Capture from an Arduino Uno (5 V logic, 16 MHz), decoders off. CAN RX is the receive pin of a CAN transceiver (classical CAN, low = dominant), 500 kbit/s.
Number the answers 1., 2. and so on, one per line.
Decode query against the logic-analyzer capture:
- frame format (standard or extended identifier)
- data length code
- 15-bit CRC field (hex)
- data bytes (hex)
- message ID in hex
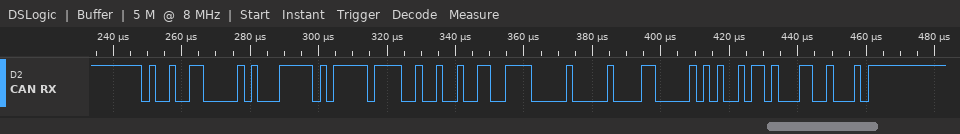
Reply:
1. standard
2. 8
3. 0x68C8
4. FD FF 24 99 E0 00 60 52
5. 0x498
